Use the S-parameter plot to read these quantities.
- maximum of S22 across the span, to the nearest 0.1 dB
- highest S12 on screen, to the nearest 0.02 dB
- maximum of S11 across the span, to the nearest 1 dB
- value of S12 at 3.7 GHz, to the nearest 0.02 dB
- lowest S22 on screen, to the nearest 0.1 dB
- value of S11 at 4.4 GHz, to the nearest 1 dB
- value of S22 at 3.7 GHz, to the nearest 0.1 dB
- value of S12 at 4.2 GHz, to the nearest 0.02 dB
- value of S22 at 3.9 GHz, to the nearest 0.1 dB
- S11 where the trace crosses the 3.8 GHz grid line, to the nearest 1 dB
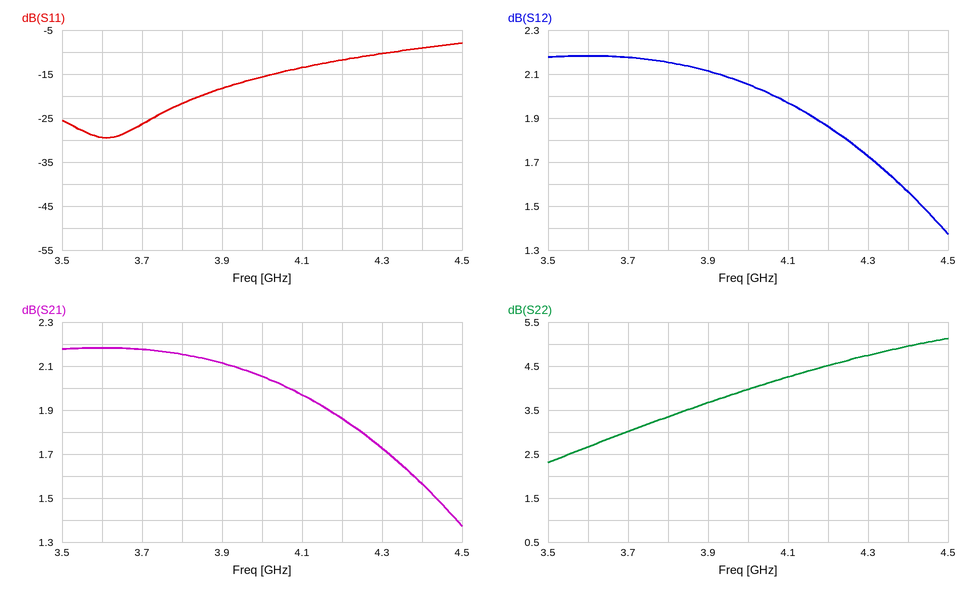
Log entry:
5.1 dB
2.18 dB
-8 dB
2.18 dB
2.3 dB
-9 dB
3.0 dB
1.86 dB
3.7 dB
-22 dB
